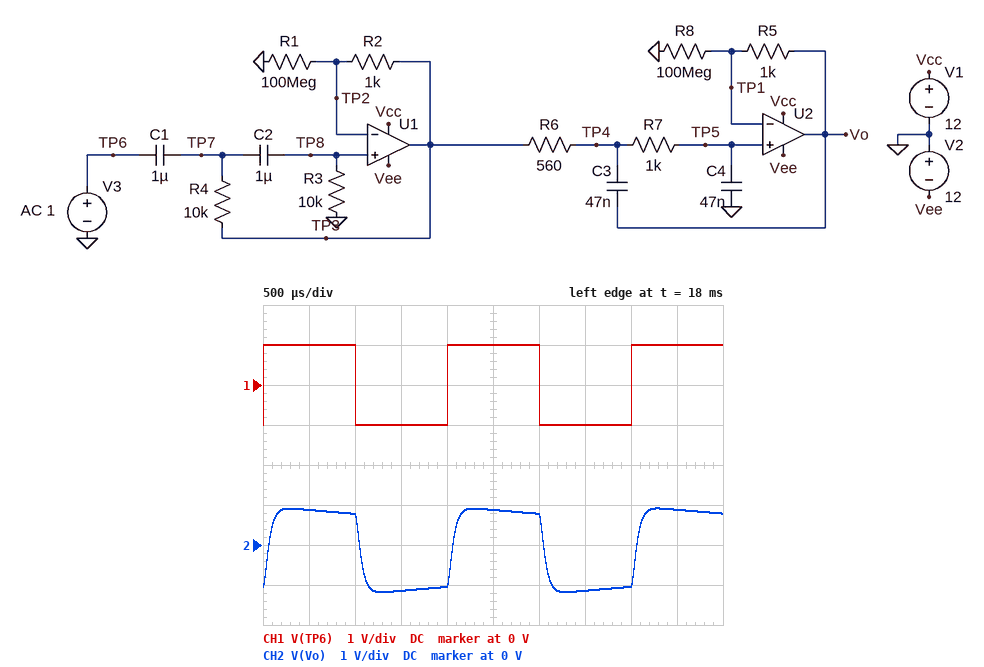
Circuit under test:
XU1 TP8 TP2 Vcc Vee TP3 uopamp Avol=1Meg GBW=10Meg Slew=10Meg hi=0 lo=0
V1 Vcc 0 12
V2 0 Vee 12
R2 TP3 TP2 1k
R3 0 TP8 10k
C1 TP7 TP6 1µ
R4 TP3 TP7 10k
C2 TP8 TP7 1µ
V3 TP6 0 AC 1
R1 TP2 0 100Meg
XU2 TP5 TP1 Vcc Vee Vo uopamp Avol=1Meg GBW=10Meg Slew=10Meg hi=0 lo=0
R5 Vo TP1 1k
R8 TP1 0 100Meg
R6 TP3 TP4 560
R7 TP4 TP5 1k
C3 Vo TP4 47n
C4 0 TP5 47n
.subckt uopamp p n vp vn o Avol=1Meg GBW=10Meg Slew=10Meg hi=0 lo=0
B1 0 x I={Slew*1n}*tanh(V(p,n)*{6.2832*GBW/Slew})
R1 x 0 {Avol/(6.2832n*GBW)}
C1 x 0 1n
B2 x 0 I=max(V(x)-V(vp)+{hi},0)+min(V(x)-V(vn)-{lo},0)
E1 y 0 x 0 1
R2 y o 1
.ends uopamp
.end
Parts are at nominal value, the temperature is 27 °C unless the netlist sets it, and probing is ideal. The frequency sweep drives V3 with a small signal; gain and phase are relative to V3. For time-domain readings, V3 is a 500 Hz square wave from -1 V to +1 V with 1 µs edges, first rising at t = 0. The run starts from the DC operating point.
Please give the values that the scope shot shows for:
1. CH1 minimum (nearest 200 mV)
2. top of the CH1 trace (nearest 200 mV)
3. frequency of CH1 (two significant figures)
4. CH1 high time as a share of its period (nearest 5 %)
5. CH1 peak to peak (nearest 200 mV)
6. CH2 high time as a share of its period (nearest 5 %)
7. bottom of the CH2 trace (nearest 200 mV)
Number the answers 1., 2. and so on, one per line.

1. -1.0 V
2. 1.0 V
3. 500 Hz
4. 50 %
5. 2.0 V
6. 50 %
7. -1.2 V
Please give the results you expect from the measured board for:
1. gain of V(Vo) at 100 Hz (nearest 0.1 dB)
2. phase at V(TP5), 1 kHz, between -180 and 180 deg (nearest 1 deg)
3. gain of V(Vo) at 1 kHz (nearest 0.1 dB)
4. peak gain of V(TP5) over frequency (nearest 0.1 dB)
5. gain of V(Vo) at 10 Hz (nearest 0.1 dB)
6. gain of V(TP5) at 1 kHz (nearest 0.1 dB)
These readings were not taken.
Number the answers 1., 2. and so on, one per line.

1. -0.2 dB
2. -24 deg
3. -0.5 dB
4. -0.1 dB
5. -11.0 dB
6. -0.5 dB
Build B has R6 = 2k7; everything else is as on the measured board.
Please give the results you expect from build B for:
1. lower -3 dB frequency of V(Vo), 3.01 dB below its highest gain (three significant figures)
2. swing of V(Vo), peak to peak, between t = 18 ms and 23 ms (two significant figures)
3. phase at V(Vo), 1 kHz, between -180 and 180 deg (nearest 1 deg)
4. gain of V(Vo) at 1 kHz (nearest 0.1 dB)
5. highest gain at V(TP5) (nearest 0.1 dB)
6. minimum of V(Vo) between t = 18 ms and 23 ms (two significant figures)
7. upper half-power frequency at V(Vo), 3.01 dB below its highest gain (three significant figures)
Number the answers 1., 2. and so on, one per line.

1. 24.0 Hz
2. 2.0 V
3. -53 deg
4. -2.5 dB
5. -0.2 dB
6. -1.1 V
7. 1.16 kHz
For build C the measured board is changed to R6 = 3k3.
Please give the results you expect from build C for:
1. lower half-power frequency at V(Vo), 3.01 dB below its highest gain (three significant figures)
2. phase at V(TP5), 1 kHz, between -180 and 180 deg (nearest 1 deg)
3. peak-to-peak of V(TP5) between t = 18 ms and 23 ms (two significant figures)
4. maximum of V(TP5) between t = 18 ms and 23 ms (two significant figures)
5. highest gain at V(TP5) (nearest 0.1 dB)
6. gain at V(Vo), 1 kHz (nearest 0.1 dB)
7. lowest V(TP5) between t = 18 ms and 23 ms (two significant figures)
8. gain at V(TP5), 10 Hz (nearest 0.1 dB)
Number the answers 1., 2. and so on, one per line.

1. 23.8 Hz
2. -59 deg
3. 1.9 V
4. 830 mV
5. -0.2 dB
6. -3.3 dB
7. -1.1 V
8. -11.0 dB
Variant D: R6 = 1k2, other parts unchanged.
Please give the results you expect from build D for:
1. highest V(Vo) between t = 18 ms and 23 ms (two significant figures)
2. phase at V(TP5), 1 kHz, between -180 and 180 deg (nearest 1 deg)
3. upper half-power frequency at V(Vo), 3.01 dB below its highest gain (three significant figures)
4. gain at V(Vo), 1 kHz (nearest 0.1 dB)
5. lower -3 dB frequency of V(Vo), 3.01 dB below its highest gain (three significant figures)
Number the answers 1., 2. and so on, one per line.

1. 900 mV
2. -34 deg
3. 2.01 kHz
4. -0.9 dB
5. 24.3 Hz
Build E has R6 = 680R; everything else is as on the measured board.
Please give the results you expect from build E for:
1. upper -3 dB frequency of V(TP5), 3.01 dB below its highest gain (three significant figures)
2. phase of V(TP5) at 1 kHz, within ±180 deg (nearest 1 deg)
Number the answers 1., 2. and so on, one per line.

1. 2.61 kHz
2. -26 deg
